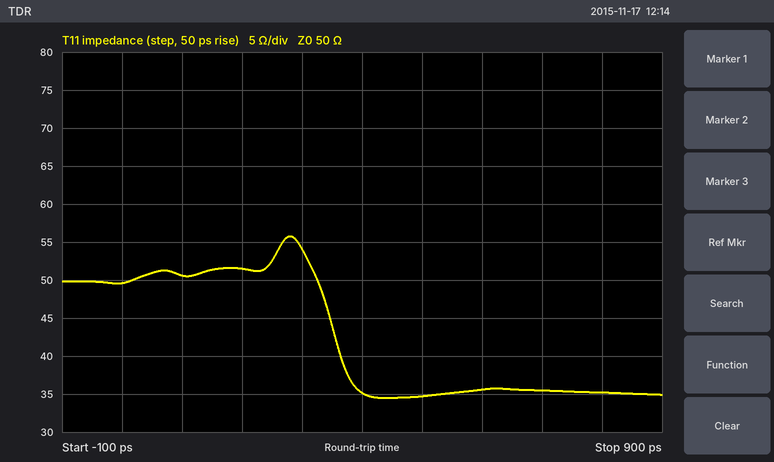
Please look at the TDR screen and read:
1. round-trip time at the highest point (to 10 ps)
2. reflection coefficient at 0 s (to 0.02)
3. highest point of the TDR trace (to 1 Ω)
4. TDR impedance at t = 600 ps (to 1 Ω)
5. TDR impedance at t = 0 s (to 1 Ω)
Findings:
280 ps
0.00
56 Ω
36 Ω
50 Ω
